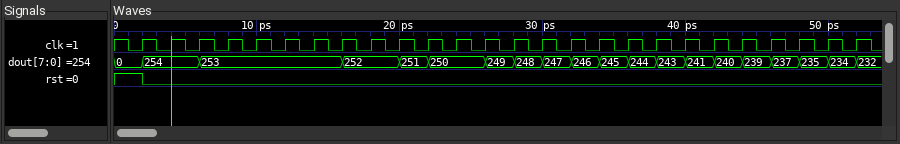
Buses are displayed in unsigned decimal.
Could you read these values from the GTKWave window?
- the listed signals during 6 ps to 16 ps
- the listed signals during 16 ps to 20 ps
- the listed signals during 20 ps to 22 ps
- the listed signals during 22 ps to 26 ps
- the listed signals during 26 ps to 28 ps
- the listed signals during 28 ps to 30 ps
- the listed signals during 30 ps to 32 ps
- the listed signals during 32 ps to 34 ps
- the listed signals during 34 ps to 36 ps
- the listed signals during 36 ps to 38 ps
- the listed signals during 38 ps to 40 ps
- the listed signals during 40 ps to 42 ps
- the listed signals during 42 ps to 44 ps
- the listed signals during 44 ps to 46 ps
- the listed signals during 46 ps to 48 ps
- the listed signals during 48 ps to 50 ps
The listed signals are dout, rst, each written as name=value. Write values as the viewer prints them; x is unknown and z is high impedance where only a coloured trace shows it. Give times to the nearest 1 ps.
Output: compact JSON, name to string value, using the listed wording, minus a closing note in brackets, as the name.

{"the listed signals during 6 ps to 16 ps": "dout=253, rst=0", "the listed signals during 16 ps to 20 ps": "dout=252, rst=0", "the listed signals during 20 ps to 22 ps": "dout=251, rst=0", "the listed signals during 22 ps to 26 ps": "dout=250, rst=0", "the listed signals during 26 ps to 28 ps": "dout=249, rst=0", "the listed signals during 28 ps to 30 ps": "dout=248, rst=0", "the listed signals during 30 ps to 32 ps": "dout=247, rst=0", "the listed signals during 32 ps to 34 ps": "dout=246, rst=0", "the listed signals during 34 ps to 36 ps": "dout=245, rst=0", "the listed signals during 36 ps to 38 ps": "dout=244, rst=0", "the listed signals during 38 ps to 40 ps": "dout=243, rst=0", "the listed signals during 40 ps to 42 ps": "dout=241, rst=0", "the listed signals during 42 ps to 44 ps": "dout=240, rst=0", "the listed signals during 44 ps to 46 ps": "dout=239, rst=0", "the listed signals during 46 ps to 48 ps": "dout=237, rst=0", "the listed signals during 48 ps to 50 ps": "dout=235, rst=0"}
